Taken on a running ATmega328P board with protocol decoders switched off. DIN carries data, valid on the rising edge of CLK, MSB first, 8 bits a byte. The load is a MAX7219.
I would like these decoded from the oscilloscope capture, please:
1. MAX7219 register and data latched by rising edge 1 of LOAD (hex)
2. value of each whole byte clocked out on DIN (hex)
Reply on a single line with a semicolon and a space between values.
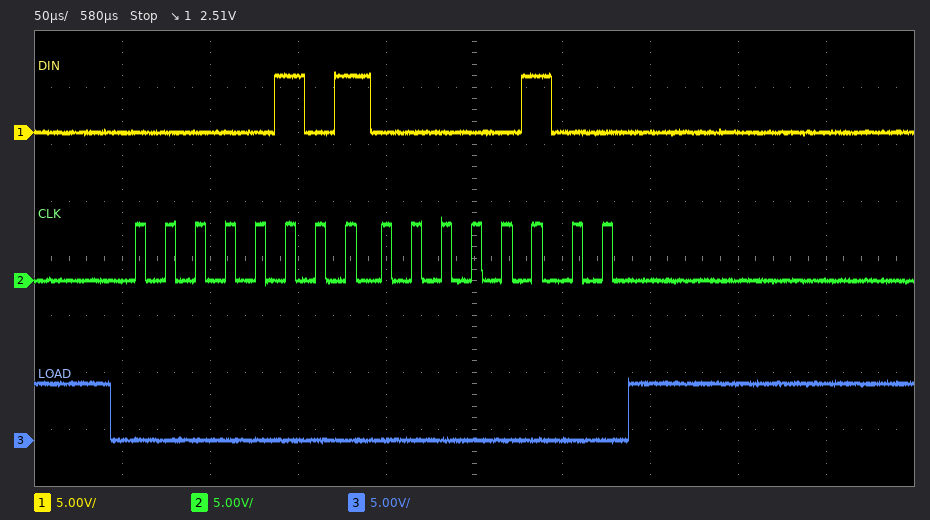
register 0x5, data 0x04; 05 04
